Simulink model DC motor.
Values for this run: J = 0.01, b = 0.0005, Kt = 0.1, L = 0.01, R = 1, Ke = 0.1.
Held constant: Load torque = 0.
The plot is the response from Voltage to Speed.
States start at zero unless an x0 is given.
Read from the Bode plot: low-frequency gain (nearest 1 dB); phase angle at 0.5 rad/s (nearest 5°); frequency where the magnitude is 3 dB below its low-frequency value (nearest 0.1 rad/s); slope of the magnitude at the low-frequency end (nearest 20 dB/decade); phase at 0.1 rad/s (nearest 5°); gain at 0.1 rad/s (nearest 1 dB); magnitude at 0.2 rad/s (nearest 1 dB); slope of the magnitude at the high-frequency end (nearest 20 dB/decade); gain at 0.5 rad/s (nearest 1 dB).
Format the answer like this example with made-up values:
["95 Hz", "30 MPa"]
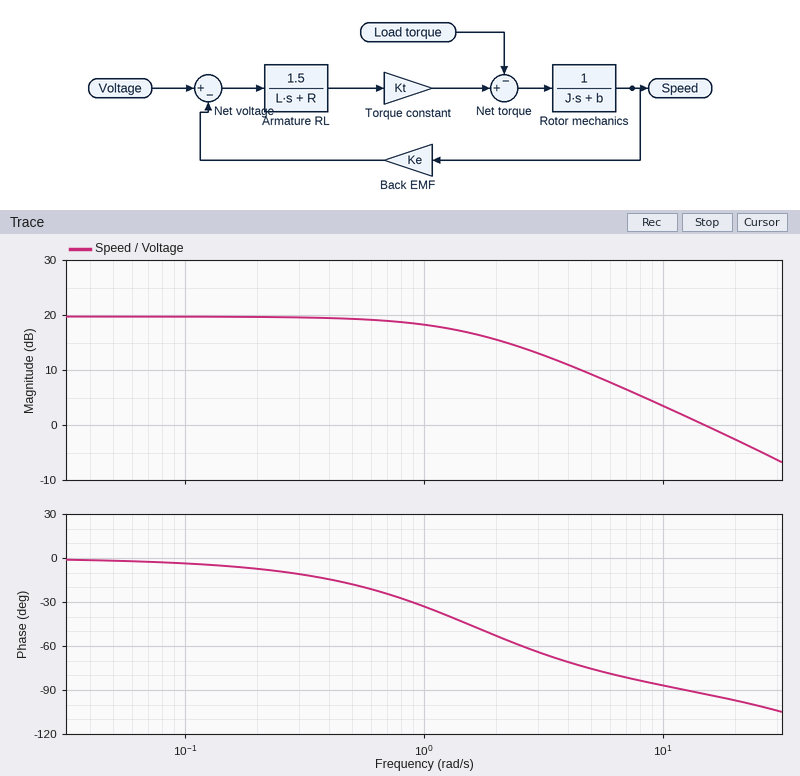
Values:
["20 dB", "-20°", "1.6 rad/s", "0 dB/decade", "-5°", "20 dB", "20 dB", "-20 dB/decade", "19 dB"]
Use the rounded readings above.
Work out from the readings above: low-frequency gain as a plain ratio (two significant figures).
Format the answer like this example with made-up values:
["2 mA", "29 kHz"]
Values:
["10"]
